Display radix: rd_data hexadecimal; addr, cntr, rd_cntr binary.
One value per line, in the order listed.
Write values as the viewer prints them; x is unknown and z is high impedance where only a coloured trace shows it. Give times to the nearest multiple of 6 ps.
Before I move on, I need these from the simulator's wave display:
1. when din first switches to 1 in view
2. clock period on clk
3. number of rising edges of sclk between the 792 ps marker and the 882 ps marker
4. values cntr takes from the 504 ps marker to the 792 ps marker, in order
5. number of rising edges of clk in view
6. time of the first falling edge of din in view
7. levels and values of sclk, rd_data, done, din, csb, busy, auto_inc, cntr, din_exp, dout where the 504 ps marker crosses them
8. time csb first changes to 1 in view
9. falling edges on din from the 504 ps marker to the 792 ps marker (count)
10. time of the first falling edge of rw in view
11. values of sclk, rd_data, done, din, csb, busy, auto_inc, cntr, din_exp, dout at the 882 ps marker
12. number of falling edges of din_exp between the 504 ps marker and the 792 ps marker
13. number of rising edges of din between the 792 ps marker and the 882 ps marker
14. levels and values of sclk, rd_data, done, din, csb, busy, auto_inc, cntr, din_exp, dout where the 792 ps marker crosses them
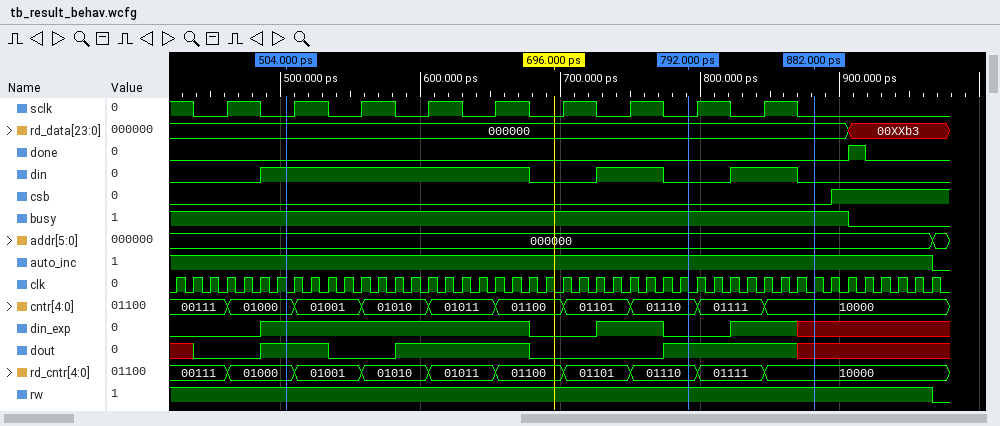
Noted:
486 ps
12 ps
2
01000, 01001, 01010, 01011, 01100, 01101, 01110
46
678 ps
sclk=0, rd_data=000000, done=0, din=1, csb=0, busy=1, auto_inc=1, cntr=01000, din_exp=1, dout=1
894 ps
2
966 ps
sclk=0, rd_data=000000, done=0, din=0, csb=0, busy=1, auto_inc=1, cntr=10000, din_exp=x, dout=x
2
1
sclk=0, rd_data=000000, done=0, din=0, csb=0, busy=1, auto_inc=1, cntr=01110, din_exp=0, dout=1
